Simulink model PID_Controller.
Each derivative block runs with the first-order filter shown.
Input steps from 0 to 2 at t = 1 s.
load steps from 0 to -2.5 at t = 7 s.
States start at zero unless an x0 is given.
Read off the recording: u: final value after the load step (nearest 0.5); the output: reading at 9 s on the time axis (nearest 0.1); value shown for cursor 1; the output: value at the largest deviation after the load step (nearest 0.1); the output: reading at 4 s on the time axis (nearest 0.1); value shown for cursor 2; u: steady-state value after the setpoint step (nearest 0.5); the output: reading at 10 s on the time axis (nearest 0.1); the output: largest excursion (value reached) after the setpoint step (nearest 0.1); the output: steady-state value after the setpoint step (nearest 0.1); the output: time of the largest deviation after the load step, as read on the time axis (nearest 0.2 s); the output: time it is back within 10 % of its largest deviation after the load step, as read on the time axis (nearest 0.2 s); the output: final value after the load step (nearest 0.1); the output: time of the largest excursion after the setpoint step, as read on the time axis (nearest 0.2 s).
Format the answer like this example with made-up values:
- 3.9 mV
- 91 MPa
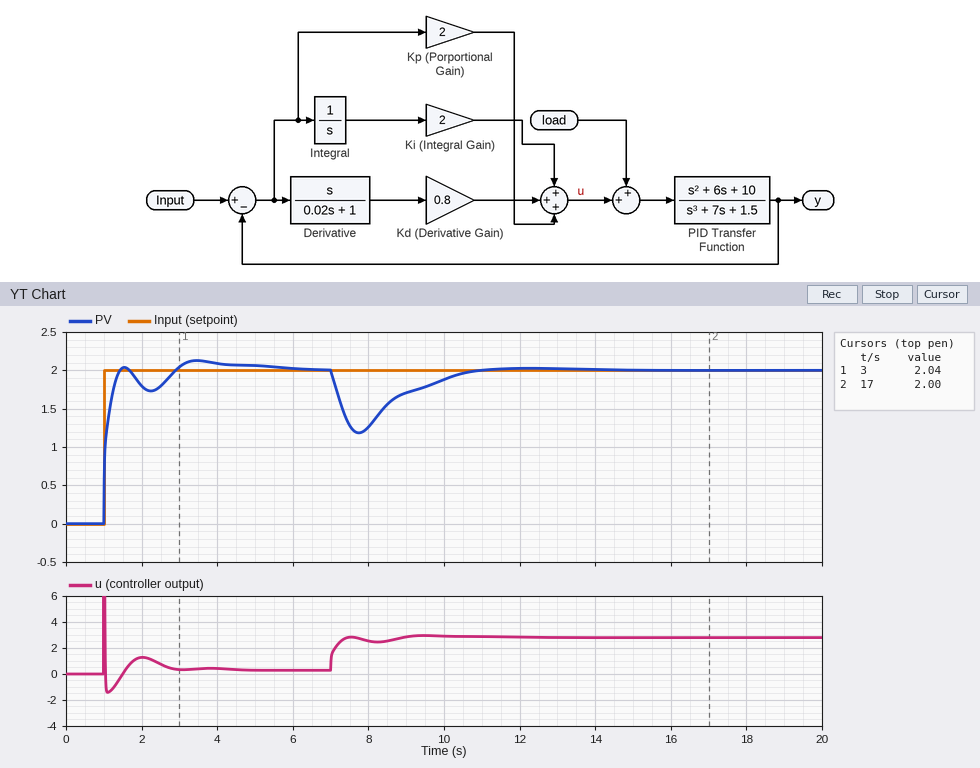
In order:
- 3.0
- 1.7
- 2.04
- 1.2
- 2.1
- 2.00
- 0.5
- 1.9
- 2.1
- 2.0
- 7.8 s
- 10.2 s
- 2.0
- 3.4 s
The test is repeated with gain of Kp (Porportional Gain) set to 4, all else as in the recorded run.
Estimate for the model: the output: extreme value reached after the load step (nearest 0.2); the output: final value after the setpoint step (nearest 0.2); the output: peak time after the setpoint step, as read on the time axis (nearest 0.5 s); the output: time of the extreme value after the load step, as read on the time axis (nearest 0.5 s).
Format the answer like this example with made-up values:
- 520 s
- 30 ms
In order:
- 1.4
- 2.0
- 1.5 s
- 7.5 s
